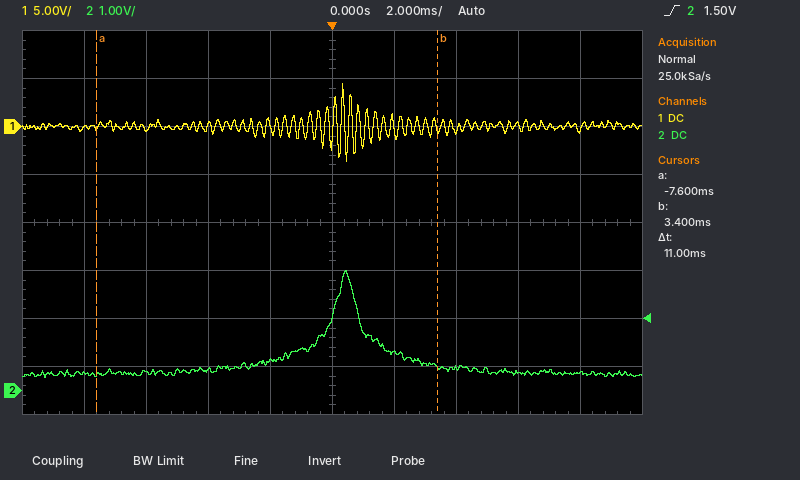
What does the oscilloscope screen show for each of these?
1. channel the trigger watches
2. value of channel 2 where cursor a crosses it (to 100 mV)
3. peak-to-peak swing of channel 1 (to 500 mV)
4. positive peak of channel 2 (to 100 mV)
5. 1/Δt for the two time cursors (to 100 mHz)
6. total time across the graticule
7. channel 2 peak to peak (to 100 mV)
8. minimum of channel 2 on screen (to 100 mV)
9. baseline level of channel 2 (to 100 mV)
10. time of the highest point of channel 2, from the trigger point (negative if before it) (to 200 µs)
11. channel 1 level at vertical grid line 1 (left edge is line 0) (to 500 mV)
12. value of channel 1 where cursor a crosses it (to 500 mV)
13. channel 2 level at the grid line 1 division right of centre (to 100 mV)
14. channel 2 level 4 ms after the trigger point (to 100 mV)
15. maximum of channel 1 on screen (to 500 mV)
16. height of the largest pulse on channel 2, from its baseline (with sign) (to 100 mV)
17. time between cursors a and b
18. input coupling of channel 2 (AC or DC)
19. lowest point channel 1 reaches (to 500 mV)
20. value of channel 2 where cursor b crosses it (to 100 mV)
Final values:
channel 2
300 mV
8.0 V
2.5 V
90.9 Hz
20 ms
2.2 V
300 mV
400 mV
+400 µs
0.0 V
0.0 V
800 mV
500 mV
4.5 V
+2.1 V
11 ms
DC
-3.5 V
500 mV
